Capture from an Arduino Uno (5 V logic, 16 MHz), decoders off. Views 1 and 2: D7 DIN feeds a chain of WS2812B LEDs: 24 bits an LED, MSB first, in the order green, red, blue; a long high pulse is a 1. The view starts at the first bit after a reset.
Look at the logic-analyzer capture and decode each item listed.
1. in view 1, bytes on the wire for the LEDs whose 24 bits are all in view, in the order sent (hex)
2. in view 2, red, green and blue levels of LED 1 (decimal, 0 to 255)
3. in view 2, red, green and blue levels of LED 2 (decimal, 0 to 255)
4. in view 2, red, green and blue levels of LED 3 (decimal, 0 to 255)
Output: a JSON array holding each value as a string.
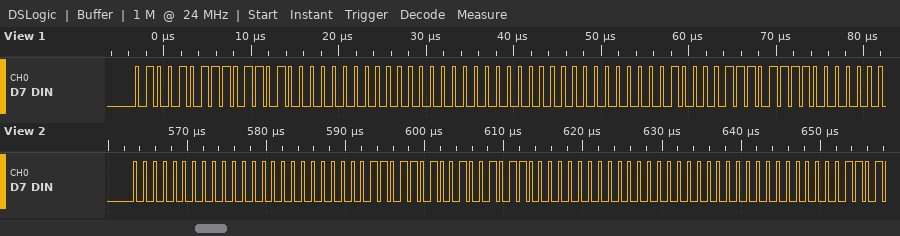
["4B B4 00 00 00 00", "0, 0, 0", "75, 218, 0", "0, 0, 0"]
